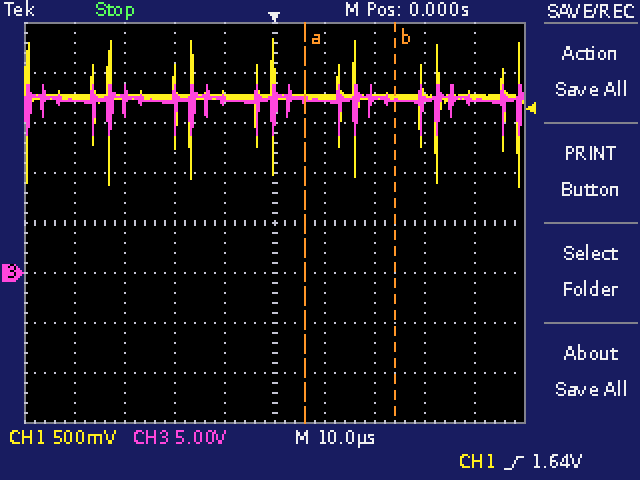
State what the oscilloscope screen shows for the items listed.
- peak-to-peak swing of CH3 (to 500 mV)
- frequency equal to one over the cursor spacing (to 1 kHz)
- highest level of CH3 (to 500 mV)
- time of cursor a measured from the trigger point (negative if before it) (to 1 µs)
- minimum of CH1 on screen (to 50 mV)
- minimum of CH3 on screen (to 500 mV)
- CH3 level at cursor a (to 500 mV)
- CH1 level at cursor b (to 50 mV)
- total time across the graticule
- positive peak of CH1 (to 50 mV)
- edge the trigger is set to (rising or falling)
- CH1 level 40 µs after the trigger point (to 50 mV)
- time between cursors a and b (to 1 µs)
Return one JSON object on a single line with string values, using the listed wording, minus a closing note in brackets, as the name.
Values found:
{"peak-to-peak swing of CH3": "5.0 V", "frequency equal to one over the cursor spacing": "56 kHz", "highest level of CH3": "19.0 V", "time of cursor a measured from the trigger point (negative if before it)": "+6 µs", "minimum of CH1 on screen": "850 mV", "minimum of CH3 on screen": "14.0 V", "CH3 level at cursor a": "17.5 V", "CH1 level at cursor b": "1.75 V", "total time across the graticule": "100 µs", "positive peak of CH1": "2.35 V", "edge the trigger is set to": "rising", "CH1 level 40 µs after the trigger point": "1.75 V", "time between cursors a and b": "18 µs"}
